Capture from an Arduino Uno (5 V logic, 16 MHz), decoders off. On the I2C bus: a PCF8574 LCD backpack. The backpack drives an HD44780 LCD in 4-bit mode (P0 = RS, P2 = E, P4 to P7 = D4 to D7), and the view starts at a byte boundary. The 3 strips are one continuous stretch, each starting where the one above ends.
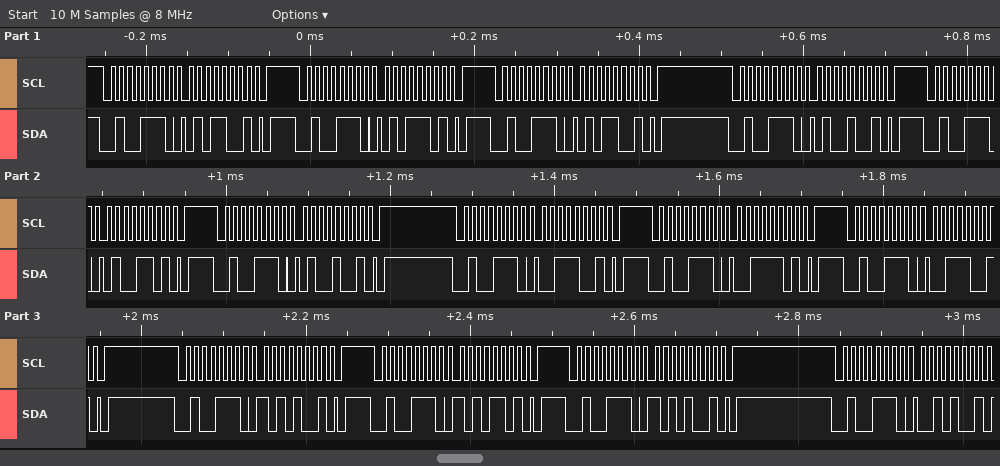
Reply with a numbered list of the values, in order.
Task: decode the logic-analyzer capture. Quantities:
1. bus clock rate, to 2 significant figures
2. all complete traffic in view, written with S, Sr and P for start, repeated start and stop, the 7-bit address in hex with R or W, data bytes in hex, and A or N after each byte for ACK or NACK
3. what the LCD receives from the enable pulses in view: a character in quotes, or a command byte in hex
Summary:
1. 100 kHz
2. S 27W A 59 A P S 27W A 5D A P S 27W A 59 A P S 27W A 49 A P S 27W A 4D A P S 27W A 49 A P S 27W A 39 A P S 27W A 3D A P S 27W A 39 A P S 27W A A9 A P S 27W A AD A P S 27W A A9 A P S 27W A 29 A
3. 'T' ':'
